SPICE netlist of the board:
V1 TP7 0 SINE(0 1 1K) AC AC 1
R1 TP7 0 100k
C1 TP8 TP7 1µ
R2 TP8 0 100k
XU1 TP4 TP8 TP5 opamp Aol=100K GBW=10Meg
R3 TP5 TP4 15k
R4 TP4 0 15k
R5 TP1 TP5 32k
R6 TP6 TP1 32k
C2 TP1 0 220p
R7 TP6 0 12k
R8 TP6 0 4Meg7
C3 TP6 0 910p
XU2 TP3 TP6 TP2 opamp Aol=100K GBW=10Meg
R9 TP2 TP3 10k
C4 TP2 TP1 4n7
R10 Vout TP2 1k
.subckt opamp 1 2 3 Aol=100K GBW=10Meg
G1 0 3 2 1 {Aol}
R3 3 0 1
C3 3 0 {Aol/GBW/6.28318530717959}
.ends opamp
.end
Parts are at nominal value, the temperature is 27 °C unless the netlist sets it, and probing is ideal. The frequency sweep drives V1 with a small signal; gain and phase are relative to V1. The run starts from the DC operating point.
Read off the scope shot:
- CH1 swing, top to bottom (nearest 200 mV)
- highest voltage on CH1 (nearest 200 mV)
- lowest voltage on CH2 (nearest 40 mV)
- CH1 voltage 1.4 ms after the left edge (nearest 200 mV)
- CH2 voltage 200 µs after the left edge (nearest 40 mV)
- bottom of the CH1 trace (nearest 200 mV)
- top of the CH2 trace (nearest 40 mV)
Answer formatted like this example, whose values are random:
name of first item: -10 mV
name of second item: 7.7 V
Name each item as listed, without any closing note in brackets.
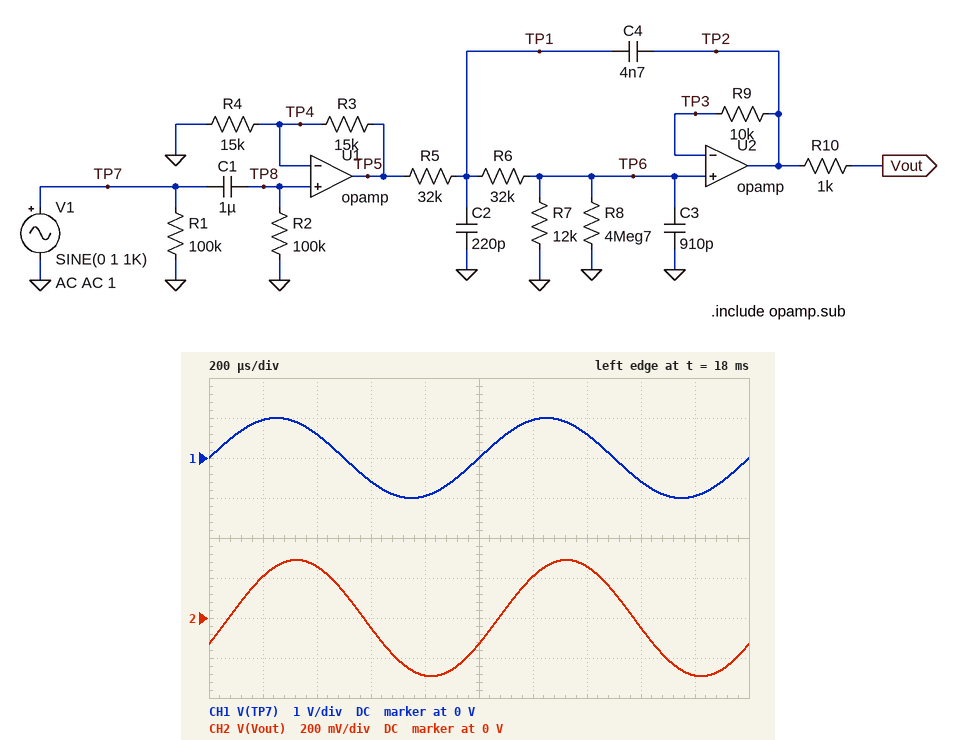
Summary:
CH1 swing, top to bottom: 2.0 V
highest voltage on CH1: 1.0 V
lowest voltage on CH2: -280 mV
CH1 voltage 1.4 ms after the left edge: 600 mV
CH2 voltage 200 µs after the left edge: 200 mV
bottom of the CH1 trace: -1.0 V
top of the CH2 trace: 280 mV
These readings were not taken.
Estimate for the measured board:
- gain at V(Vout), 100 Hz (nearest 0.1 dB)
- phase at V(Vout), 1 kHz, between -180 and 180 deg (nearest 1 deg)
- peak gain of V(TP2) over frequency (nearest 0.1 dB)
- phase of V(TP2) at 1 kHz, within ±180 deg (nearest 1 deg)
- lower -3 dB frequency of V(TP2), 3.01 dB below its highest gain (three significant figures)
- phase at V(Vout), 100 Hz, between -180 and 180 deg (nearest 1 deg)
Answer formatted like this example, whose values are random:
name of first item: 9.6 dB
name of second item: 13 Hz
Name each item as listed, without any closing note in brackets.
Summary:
gain at V(Vout), 100 Hz: -10.0 dB
phase at V(Vout), 1 kHz, between -180 and 180 deg: -26 deg
peak gain of V(TP2) over frequency: -10.0 dB
phase of V(TP2) at 1 kHz, within ±180 deg: -26 deg
lower -3 dB frequency of V(TP2), 3.01 dB below its highest gain: 1.59 Hz
phase at V(Vout), 100 Hz, between -180 and 180 deg: -2 deg
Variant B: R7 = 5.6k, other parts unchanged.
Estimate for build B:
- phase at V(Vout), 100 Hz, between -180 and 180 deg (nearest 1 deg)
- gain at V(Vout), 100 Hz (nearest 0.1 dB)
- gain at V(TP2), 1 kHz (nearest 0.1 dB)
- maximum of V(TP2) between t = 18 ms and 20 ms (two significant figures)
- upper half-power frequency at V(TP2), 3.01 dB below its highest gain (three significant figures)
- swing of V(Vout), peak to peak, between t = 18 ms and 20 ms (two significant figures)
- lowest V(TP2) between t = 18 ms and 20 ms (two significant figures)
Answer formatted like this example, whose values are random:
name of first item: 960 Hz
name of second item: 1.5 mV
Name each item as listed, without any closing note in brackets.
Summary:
phase at V(Vout), 100 Hz, between -180 and 180 deg: -2 deg
gain at V(Vout), 100 Hz: -15.9 dB
gain at V(TP2), 1 kHz: -16.7 dB
maximum of V(TP2) between t = 18 ms and 20 ms: 150 mV
upper half-power frequency at V(TP2), 3.01 dB below its highest gain: 2.19 kHz
swing of V(Vout), peak to peak, between t = 18 ms and 20 ms: 290 mV
lowest V(TP2) between t = 18 ms and 20 ms: -150 mV
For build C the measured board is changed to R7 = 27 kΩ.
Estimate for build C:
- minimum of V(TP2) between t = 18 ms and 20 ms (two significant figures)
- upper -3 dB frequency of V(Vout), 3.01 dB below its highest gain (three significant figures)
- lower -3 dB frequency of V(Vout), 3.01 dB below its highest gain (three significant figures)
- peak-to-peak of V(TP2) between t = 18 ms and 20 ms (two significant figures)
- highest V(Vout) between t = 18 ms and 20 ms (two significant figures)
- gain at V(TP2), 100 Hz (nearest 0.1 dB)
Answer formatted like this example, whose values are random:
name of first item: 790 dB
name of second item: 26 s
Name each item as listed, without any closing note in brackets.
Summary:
minimum of V(TP2) between t = 18 ms and 20 ms: -560 mV
upper -3 dB frequency of V(Vout), 3.01 dB below its highest gain: 2.73 kHz
lower -3 dB frequency of V(Vout), 3.01 dB below its highest gain: 1.59 Hz
peak-to-peak of V(TP2) between t = 18 ms and 20 ms: 1.1 V
highest V(Vout) between t = 18 ms and 20 ms: 560 mV
gain at V(TP2), 100 Hz: -4.6 dB
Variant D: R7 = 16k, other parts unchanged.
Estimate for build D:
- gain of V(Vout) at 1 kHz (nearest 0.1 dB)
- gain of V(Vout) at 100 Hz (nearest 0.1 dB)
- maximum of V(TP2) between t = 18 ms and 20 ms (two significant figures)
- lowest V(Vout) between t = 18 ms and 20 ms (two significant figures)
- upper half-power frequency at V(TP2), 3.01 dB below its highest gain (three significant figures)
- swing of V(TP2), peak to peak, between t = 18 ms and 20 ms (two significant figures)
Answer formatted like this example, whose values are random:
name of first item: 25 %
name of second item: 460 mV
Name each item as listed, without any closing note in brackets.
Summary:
gain of V(Vout) at 1 kHz: -8.6 dB
gain of V(Vout) at 100 Hz: -8.0 dB
maximum of V(TP2) between t = 18 ms and 20 ms: 370 mV
lowest V(Vout) between t = 18 ms and 20 ms: -370 mV
upper half-power frequency at V(TP2), 3.01 dB below its highest gain: 2.47 kHz
swing of V(TP2), peak to peak, between t = 18 ms and 20 ms: 740 mV
